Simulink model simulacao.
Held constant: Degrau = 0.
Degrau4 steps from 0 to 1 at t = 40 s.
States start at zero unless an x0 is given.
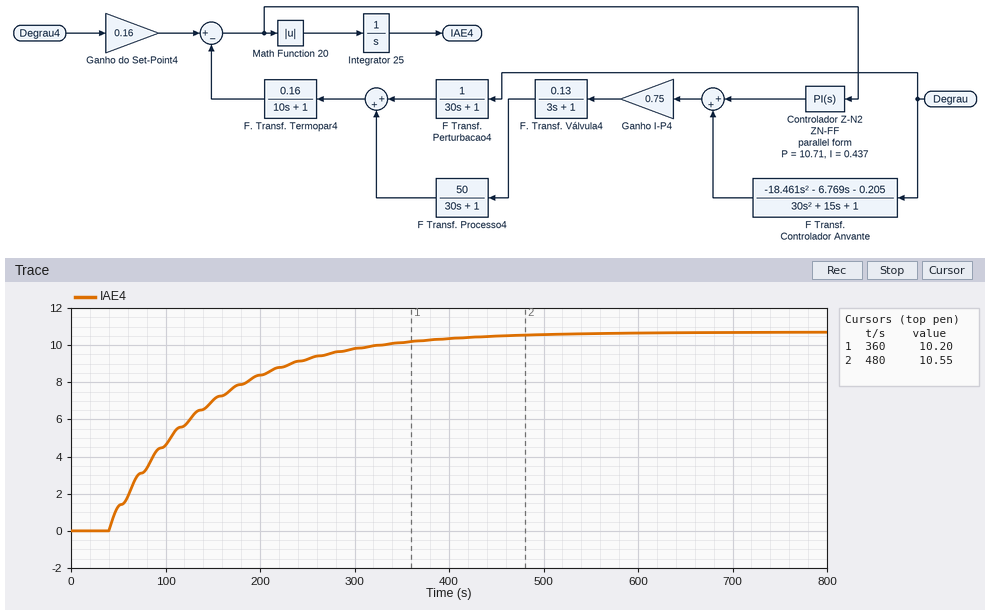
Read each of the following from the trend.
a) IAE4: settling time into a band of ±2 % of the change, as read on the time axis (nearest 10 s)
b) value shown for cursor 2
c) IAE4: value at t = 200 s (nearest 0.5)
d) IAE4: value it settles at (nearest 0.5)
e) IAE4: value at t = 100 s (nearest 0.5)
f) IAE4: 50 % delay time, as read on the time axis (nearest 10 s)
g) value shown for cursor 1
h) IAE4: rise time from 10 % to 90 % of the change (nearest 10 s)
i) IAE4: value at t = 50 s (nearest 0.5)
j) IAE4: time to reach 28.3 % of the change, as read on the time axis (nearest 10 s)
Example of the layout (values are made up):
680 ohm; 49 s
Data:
460 s; 10.55; 8.5; 10.5; 4.5; 110 s; 10.20; 230 s; 1.5; 70 s
